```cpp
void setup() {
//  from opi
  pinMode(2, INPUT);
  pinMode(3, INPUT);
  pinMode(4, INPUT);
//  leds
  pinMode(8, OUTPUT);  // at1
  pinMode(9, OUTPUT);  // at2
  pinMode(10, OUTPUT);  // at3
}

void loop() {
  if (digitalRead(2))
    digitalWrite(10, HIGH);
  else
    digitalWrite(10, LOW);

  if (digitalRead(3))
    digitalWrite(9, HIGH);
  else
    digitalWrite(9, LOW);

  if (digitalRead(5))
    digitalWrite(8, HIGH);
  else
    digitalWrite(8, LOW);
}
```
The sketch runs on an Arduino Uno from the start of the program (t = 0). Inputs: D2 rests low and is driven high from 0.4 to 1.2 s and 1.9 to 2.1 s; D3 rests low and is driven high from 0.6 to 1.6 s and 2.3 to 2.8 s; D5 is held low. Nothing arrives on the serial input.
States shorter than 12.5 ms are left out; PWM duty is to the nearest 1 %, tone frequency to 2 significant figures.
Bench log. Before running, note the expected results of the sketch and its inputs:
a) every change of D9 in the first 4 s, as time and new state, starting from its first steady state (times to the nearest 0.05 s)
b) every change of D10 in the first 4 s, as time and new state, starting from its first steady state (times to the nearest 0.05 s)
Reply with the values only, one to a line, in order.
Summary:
0 s low; 0.6 s high; 1.6 s low; 2.3 s high; 2.8 s low
0 s low; 0.4 s high; 1.2 s low; 1.9 s high; 2.1 s low
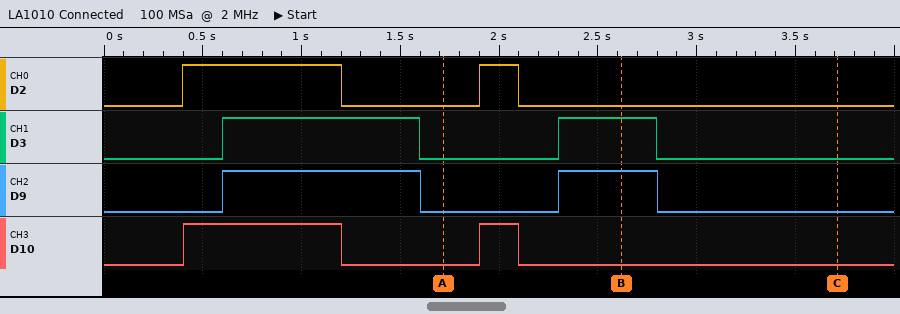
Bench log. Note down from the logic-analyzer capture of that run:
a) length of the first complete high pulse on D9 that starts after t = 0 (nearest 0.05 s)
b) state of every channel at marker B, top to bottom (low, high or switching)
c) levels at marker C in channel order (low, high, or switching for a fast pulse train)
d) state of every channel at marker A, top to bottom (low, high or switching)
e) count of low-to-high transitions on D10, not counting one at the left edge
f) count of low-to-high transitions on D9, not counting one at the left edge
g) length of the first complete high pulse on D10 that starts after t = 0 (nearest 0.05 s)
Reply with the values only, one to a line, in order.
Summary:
1.00 s
D2 low, D3 high, D9 high, D10 low
D2 low, D3 low, D9 low, D10 low
D2 low, D3 low, D9 low, D10 low
2
2
0.80 s
